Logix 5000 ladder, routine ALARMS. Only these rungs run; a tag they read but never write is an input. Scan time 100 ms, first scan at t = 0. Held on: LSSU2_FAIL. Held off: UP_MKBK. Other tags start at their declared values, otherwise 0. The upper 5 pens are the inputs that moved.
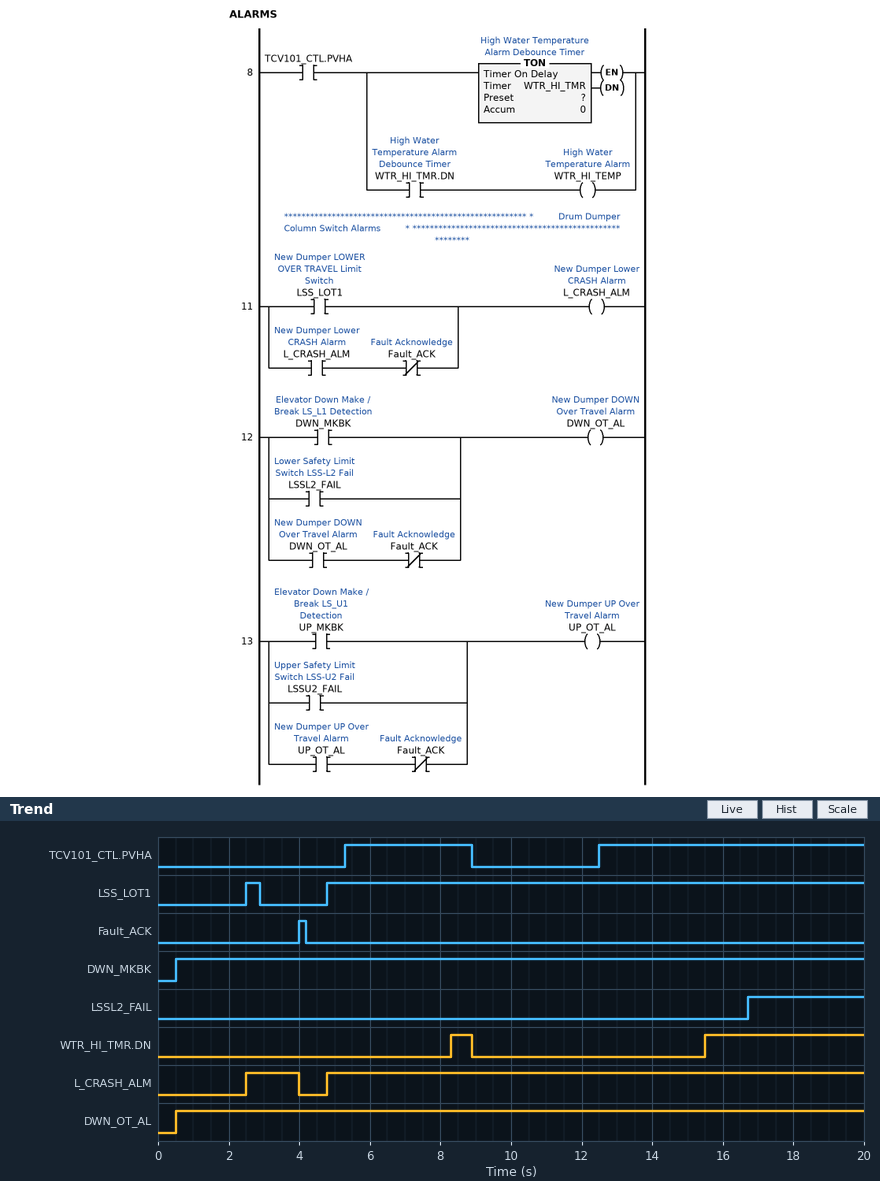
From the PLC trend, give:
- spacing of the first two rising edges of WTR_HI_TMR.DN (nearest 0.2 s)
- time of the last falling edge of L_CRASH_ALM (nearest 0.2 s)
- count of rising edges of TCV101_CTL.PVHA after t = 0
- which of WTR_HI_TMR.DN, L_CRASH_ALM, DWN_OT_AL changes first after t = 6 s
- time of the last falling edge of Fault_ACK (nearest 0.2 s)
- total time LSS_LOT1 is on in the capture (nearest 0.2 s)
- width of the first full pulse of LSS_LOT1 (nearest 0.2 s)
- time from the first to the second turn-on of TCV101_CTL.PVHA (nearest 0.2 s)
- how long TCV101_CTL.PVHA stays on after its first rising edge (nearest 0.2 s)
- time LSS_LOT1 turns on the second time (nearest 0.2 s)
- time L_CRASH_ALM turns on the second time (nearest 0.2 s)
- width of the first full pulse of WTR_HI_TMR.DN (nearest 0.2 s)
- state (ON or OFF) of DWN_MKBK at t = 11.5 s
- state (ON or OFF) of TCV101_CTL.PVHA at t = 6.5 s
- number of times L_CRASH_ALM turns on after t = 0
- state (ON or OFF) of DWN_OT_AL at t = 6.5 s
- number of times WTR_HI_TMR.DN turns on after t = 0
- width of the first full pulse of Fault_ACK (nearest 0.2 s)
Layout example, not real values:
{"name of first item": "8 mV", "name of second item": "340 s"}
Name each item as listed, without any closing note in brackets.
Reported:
{"spacing of the first two rising edges of WTR_HI_TMR.DN": "7.2 s", "time of the last falling edge of L_CRASH_ALM": "4.0 s", "count of rising edges of TCV101_CTL.PVHA after t = 0": "2", "which of WTR_HI_TMR.DN, L_CRASH_ALM, DWN_OT_AL changes first after t = 6 s": "WTR_HI_TMR.DN", "time of the last falling edge of Fault_ACK": "4.2 s", "total time LSS_LOT1 is on in the capture": "15.6 s", "width of the first full pulse of LSS_LOT1": "0.4 s", "time from the first to the second turn-on of TCV101_CTL.PVHA": "7.2 s", "how long TCV101_CTL.PVHA stays on after its first rising edge": "3.6 s", "time LSS_LOT1 turns on the second time": "4.8 s", "time L_CRASH_ALM turns on the second time": "4.8 s", "width of the first full pulse of WTR_HI_TMR.DN": "0.6 s", "state (ON or OFF) of DWN_MKBK at t = 11.5 s": "ON", "state (ON or OFF) of TCV101_CTL.PVHA at t = 6.5 s": "ON", "number of times L_CRASH_ALM turns on after t = 0": "2", "state (ON or OFF) of DWN_OT_AL at t = 6.5 s": "ON", "number of times WTR_HI_TMR.DN turns on after t = 0": "2", "width of the first full pulse of Fault_ACK": "0.2 s"}
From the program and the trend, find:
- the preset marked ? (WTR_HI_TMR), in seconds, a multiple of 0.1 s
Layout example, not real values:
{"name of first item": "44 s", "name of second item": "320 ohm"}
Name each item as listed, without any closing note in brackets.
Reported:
{"the preset marked ? (WTR_HI_TMR), in seconds, a multiple of 0.1 s": "3.0 s"}
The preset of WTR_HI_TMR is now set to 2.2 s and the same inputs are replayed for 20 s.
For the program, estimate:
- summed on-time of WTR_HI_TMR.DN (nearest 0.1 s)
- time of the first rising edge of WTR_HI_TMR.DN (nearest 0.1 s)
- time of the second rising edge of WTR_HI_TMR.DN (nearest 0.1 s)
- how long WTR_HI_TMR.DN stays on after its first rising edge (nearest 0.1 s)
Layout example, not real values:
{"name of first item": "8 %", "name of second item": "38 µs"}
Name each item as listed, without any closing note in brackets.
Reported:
{"summed on-time of WTR_HI_TMR.DN": "6.7 s", "time of the first rising edge of WTR_HI_TMR.DN": "7.5 s", "time of the second rising edge of WTR_HI_TMR.DN": "14.7 s", "how long WTR_HI_TMR.DN stays on after its first rising edge": "1.4 s"}
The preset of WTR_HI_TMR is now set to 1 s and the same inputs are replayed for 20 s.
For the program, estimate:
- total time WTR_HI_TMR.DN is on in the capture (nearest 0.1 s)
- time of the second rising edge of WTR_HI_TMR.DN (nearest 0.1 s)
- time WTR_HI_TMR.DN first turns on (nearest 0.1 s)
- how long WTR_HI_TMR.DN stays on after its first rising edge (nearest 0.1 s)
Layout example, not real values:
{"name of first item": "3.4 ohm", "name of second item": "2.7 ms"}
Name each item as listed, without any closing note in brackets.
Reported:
{"total time WTR_HI_TMR.DN is on in the capture": "9.1 s", "time of the second rising edge of WTR_HI_TMR.DN": "13.5 s", "time WTR_HI_TMR.DN first turns on": "6.3 s", "how long WTR_HI_TMR.DN stays on after its first rising edge": "2.6 s"}
